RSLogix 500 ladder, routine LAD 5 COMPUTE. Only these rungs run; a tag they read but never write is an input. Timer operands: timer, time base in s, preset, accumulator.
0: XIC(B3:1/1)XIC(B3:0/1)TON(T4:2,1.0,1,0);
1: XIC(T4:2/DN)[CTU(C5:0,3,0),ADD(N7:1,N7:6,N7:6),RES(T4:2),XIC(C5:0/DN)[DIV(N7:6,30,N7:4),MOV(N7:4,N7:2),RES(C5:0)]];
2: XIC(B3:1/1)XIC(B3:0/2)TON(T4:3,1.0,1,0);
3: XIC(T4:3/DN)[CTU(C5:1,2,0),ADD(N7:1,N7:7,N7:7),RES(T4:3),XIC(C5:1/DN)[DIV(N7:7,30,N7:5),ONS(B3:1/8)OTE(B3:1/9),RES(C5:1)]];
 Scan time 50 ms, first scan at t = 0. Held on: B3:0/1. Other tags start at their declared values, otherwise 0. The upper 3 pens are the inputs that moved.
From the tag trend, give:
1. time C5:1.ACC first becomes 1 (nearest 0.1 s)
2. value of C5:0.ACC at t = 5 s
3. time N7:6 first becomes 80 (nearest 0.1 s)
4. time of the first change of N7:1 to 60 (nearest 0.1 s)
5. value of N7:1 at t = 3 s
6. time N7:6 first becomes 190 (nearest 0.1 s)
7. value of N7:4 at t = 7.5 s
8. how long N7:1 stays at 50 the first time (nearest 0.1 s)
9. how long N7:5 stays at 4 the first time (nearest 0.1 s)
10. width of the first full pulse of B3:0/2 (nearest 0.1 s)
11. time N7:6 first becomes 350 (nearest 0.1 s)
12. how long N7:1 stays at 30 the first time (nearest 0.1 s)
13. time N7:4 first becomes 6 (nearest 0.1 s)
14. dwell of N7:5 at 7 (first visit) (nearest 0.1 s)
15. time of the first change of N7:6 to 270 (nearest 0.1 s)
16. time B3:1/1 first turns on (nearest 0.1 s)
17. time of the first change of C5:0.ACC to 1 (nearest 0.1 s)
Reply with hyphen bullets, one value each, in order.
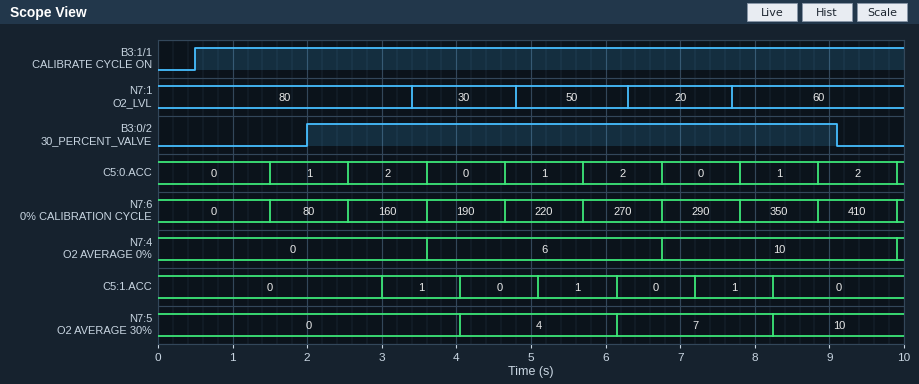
- 3.0 s
- 1
- 1.5 s
- 7.7 s
- 80
- 3.6 s
- 10
- 1.5 s
- 2.1 s
- 7.1 s
- 7.8 s
- 1.4 s
- 3.6 s
- 2.1 s
- 5.7 s
- 0.5 s
- 1.5 s
